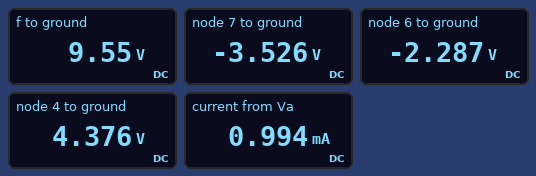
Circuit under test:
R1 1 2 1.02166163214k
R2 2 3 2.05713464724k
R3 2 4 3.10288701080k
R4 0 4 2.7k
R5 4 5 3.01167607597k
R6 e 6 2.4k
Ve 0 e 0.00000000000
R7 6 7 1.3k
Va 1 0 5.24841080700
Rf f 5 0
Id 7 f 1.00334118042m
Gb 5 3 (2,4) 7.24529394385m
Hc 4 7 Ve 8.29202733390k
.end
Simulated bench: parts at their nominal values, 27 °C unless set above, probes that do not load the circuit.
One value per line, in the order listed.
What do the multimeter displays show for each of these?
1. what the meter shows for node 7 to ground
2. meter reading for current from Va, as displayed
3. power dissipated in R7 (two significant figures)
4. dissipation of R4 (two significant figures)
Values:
-3.526 V
0.994 mA
1.2 mW
7.1 mW
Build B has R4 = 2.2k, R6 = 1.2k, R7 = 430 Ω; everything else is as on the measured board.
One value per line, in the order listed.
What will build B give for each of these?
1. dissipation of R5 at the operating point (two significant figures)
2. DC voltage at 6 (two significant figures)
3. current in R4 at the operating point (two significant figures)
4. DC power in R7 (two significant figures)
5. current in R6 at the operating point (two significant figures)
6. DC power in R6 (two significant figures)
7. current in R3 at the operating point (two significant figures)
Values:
15 mW
-700 mV
1.8 mA
150 µW
580 µA
410 µW
72 µA
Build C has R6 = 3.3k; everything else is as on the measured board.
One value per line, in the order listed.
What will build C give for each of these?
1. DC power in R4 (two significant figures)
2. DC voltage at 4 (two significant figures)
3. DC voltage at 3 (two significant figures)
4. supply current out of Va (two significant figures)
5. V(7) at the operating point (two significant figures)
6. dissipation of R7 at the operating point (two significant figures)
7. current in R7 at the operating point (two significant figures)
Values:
7.8 mW
4.6 V
2.8 V
770 µA
-5.7 V
2.0 mW
1.2 mA
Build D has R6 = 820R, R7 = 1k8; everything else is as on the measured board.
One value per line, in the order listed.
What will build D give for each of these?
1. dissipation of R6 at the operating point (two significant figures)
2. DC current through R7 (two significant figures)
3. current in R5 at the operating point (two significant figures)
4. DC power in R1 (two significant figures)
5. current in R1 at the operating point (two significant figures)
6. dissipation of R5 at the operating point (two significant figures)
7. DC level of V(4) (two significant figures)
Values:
460 µW
750 µA
1.9 mA
1.4 mW
1.2 mA
11 mW
4.2 V
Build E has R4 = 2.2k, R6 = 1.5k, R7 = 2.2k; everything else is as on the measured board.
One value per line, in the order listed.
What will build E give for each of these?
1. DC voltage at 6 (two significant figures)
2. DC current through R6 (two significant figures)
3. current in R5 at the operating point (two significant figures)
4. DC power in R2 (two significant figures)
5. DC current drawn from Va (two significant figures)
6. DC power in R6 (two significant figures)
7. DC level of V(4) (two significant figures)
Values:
-1.3 V
890 µA
2.0 mA
3.9 mW
1.3 mA
1.2 mW
4.1 V
